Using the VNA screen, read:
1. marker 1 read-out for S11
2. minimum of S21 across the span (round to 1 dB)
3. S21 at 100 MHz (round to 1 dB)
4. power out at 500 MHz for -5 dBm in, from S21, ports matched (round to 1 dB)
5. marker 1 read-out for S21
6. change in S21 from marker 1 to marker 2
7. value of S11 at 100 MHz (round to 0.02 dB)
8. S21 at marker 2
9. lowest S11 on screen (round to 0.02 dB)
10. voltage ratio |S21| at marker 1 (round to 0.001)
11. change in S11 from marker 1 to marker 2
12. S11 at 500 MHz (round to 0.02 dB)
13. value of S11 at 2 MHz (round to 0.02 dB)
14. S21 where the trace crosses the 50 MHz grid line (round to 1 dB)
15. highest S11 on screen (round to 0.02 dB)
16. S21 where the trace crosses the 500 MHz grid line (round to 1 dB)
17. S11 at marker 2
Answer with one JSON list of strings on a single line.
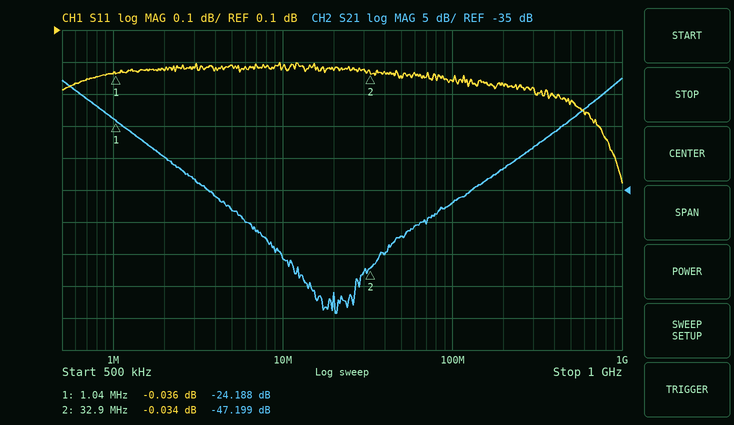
["-0.036 dB", "-54 dB", "-37 dB", "-29 dBm", "-24.188 dB", "-23.011 dB", "-0.06 dB", "-47.199 dB", "-0.38 dB", "0.062", "0.002 dB", "-0.12 dB", "-0.02 dB", "-42 dB", "0.00 dB", "-24 dB", "-0.034 dB"]
